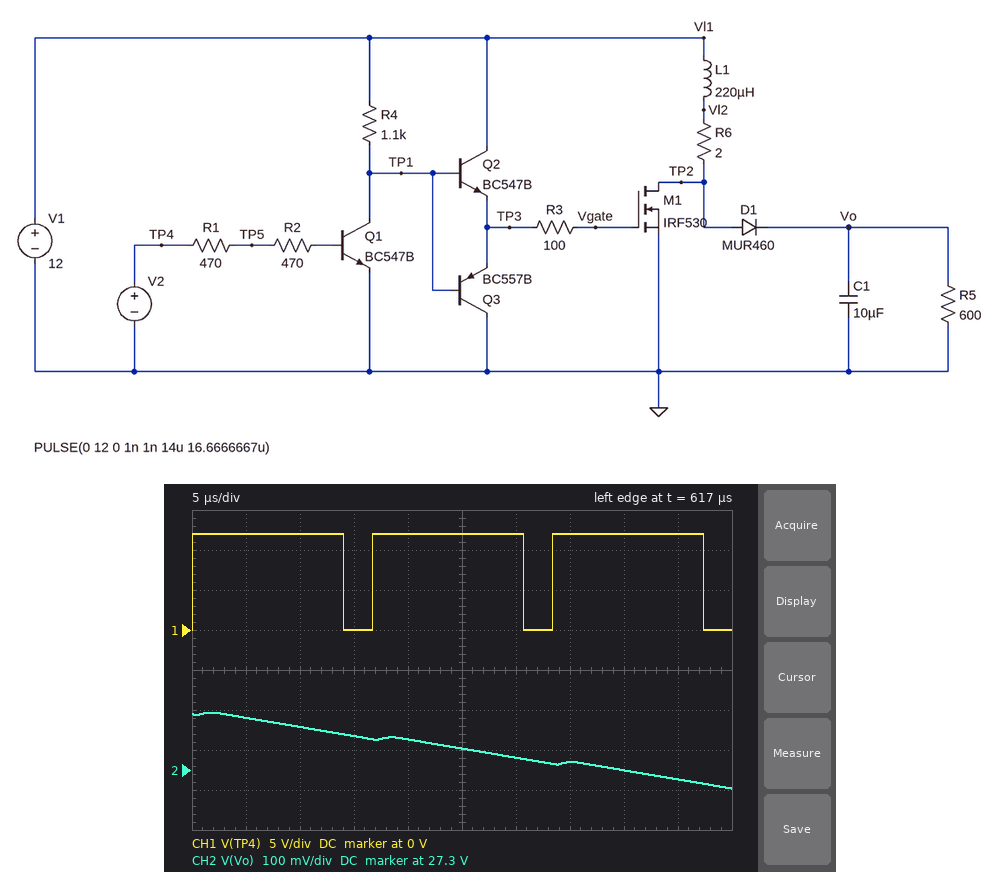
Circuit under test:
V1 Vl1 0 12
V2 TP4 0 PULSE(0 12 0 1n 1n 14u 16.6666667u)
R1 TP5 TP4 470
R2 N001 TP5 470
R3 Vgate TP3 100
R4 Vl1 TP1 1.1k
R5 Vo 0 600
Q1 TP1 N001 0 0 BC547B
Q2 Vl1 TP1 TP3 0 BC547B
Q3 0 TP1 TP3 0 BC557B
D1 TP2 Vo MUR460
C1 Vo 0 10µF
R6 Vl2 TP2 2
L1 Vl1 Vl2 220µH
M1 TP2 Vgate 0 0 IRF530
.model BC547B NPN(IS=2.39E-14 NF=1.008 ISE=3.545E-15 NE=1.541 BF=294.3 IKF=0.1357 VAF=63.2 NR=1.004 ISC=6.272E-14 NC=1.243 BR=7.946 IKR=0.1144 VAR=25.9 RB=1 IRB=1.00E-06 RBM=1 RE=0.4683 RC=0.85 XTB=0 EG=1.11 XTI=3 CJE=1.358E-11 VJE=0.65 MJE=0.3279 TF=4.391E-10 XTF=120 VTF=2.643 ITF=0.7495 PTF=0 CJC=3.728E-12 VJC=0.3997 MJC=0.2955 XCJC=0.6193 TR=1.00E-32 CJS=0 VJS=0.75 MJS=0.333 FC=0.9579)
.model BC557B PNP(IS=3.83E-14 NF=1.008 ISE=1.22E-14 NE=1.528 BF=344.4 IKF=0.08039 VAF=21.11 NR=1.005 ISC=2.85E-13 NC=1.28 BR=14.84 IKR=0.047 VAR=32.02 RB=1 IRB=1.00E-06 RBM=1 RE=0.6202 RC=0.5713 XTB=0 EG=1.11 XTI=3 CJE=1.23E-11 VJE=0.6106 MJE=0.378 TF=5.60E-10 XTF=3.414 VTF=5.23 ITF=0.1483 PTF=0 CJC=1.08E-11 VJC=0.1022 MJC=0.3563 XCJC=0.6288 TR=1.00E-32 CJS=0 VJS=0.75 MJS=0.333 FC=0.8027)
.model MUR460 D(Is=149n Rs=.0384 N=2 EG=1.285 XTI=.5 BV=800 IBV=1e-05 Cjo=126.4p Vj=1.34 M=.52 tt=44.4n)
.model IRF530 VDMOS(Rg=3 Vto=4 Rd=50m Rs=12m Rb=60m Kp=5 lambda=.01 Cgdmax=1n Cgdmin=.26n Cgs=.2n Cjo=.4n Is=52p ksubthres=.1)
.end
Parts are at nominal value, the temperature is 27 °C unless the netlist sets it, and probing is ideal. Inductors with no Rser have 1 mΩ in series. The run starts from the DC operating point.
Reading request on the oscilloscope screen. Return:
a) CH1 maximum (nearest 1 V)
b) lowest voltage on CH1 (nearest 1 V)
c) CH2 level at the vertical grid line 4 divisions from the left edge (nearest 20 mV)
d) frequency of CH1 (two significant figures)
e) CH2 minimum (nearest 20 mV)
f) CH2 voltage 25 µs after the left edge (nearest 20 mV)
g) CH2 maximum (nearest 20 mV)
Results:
12 V
0 V
27.38 V
60 kHz
27.26 V
27.36 V
27.44 V
